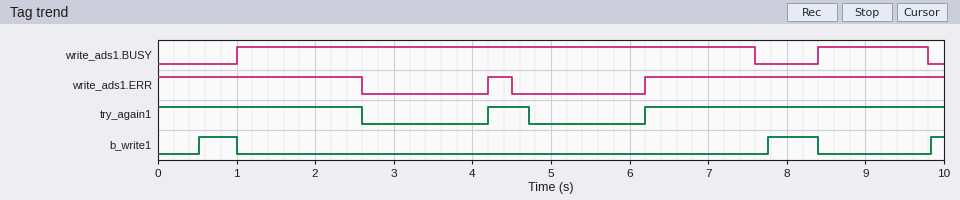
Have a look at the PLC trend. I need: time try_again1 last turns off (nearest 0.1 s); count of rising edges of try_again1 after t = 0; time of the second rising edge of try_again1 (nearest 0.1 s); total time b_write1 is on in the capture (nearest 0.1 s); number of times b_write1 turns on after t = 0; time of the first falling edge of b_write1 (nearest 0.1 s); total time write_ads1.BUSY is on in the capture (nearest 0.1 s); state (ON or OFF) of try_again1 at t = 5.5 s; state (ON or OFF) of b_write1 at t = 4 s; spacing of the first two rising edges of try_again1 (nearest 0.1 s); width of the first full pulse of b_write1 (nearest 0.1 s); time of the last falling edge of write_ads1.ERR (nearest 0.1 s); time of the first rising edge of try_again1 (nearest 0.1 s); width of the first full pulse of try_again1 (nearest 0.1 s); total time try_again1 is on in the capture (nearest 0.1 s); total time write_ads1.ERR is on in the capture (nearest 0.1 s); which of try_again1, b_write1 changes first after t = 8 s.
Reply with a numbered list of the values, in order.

1. 4.7 s
2. 2
3. 6.2 s
4. 1.3 s
5. 3
6. 1.0 s
7. 8.0 s
8. OFF
9. OFF
10. 2.0 s
11. 0.5 s
12. 4.5 s
13. 4.2 s
14. 0.5 s
15. 6.9 s
16. 6.7 s
17. b_write1
